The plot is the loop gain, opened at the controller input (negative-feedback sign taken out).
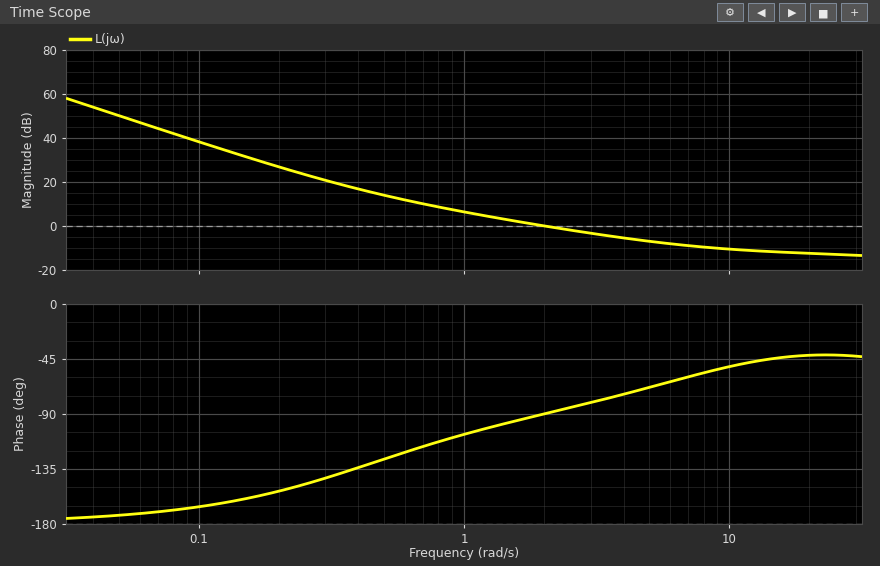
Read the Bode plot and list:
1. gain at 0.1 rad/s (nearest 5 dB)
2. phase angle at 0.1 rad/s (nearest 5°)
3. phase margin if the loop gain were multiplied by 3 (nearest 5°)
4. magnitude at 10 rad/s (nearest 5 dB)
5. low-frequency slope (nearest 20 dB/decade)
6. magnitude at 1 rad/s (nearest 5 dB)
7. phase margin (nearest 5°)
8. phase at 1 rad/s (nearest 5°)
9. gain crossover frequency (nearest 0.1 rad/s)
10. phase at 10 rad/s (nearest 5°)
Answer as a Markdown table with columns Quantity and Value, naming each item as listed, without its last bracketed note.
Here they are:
| Quantity | Value |
|---|---|
| gain at 0.1 rad/s | 40 dB |
| phase angle at 0.1 rad/s | -165° |
| phase margin if the loop gain were multiplied by 3 | 125° |
| magnitude at 10 rad/s | -10 dB |
| low-frequency slope | -40 dB/decade |
| magnitude at 1 rad/s | 5 dB |
| phase margin | 90° |
| phase at 1 rad/s | -105° |
| gain crossover frequency | 2.0 rad/s |
| phase at 10 rad/s | -50° |
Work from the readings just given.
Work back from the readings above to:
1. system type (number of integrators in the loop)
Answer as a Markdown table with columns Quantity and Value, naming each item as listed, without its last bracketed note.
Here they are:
| Quantity | Value |
|---|---|
| system type | 2 |
